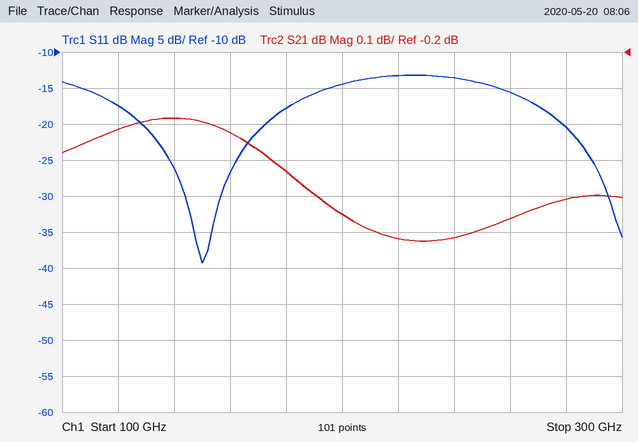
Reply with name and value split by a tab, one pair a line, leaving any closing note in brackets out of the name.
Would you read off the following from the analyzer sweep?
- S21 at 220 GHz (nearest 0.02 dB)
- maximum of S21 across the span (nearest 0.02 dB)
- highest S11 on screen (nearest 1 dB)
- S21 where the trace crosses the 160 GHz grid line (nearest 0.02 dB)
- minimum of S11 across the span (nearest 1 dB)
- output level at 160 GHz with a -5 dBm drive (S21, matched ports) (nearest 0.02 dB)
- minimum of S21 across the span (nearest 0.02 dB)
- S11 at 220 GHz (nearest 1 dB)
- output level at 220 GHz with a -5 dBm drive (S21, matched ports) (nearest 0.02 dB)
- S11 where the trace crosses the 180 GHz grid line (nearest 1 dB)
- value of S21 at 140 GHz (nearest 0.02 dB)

S21 at 220 GHz	-0.72 dB
maximum of S21 across the span	-0.38 dB
highest S11 on screen	-13 dB
S21 where the trace crosses the 160 GHz grid line	-0.42 dB
minimum of S11 across the span	-39 dB
output level at 160 GHz with a -5 dBm drive (S21, matched ports)	-5.42 dBm
minimum of S21 across the span	-0.72 dB
S11 at 220 GHz	-13 dB
output level at 220 GHz with a -5 dBm drive (S21, matched ports)	-5.72 dBm
S11 where the trace crosses the 180 GHz grid line	-18 dB
value of S21 at 140 GHz	-0.38 dB
